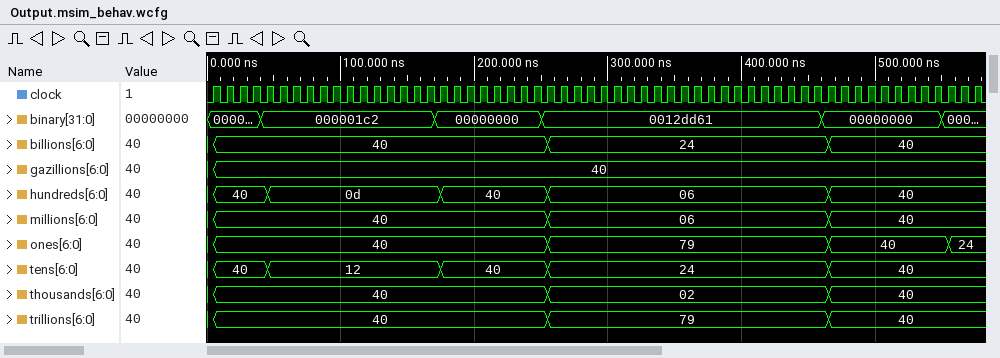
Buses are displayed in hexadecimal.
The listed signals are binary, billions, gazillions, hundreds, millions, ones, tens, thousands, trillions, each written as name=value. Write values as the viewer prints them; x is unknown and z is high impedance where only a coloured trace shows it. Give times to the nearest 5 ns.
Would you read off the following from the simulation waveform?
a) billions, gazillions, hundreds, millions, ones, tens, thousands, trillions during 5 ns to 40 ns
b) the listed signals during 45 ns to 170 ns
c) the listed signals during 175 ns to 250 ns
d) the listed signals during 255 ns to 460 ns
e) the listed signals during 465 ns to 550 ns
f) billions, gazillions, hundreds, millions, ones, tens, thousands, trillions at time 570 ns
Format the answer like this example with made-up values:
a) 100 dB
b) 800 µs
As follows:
a) billions=40, gazillions=40, hundreds=40, millions=40, ones=40, tens=40, thousands=40, trillions=40
b) binary=000001c2, billions=40, gazillions=40, hundreds=0d, millions=40, ones=40, tens=12, thousands=40, trillions=40
c) binary=00000000, billions=40, gazillions=40, hundreds=40, millions=40, ones=40, tens=40, thousands=40, trillions=40
d) binary=0012dd61, billions=24, gazillions=40, hundreds=06, millions=06, ones=79, tens=24, thousands=02, trillions=79
e) binary=00000000, billions=40, gazillions=40, hundreds=40, millions=40, ones=40, tens=40, thousands=40, trillions=40
f) billions=40, gazillions=40, hundreds=40, millions=40, ones=24, tens=40, thousands=40, trillions=40
